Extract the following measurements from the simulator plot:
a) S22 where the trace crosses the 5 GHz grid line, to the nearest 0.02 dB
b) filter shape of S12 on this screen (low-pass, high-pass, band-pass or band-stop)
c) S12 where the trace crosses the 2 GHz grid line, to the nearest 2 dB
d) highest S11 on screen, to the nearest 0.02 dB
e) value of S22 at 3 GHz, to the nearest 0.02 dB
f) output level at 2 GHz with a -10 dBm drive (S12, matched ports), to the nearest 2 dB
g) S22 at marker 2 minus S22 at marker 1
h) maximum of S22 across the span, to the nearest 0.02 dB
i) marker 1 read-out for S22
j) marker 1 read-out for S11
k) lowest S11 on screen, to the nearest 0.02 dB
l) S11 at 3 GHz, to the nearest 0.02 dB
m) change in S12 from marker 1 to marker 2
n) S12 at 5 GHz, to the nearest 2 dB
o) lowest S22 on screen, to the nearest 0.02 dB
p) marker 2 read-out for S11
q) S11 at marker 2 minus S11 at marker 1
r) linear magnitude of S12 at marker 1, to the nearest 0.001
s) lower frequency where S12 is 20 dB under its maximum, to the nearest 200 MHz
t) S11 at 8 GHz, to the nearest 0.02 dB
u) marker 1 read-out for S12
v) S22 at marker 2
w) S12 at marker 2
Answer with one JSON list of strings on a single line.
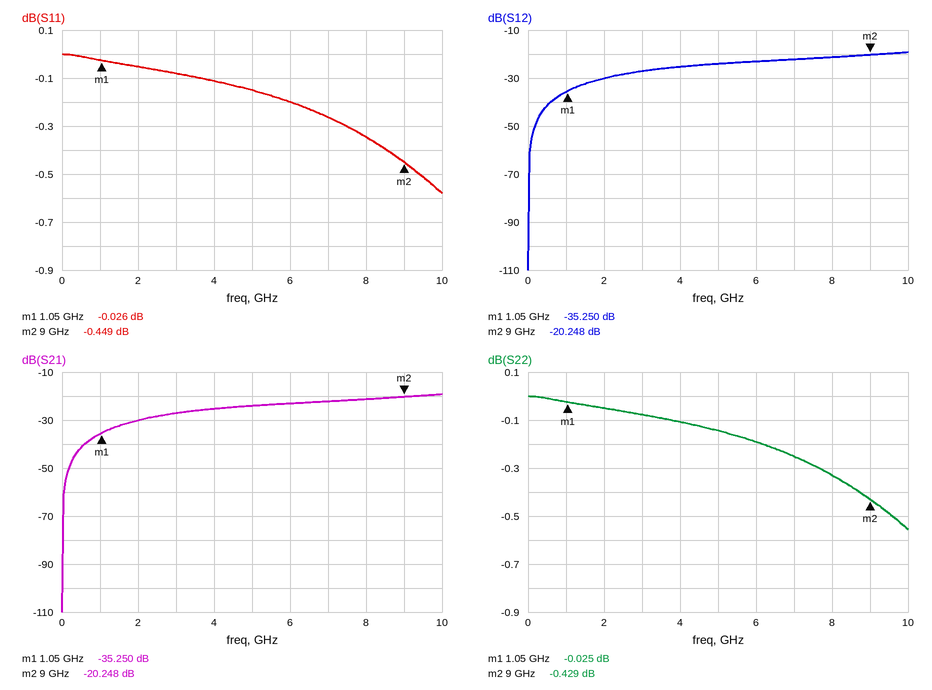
["-0.14 dB", "high-pass", "-30 dB", "0.00 dB", "-0.08 dB", "-40 dBm", "-0.404 dB", "0.00 dB", "-0.025 dB", "-0.026 dB", "-0.58 dB", "-0.08 dB", "15.002 dB", "-24 dB", "-0.56 dB", "-0.449 dB", "-0.423 dB", "0.017", "600 MHz", "-0.34 dB", "-35.250 dB", "-0.429 dB", "-20.248 dB"]
